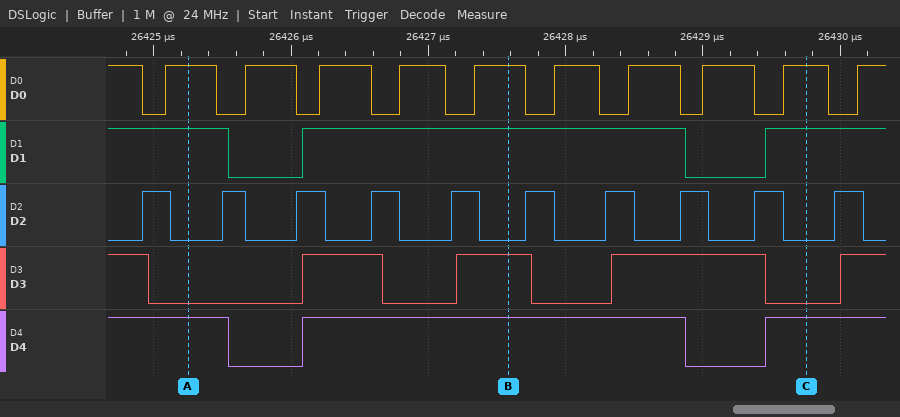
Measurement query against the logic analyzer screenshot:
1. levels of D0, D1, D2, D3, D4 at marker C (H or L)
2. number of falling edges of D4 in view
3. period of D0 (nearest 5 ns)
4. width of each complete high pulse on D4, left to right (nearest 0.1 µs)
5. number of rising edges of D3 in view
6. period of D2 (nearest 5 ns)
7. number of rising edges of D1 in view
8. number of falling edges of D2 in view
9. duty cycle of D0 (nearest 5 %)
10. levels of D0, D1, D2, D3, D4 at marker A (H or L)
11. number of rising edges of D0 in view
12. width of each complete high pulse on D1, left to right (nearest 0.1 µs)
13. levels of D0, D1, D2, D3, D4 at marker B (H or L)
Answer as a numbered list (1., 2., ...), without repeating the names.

1. D0=H, D1=H, D2=L, D3=L, D4=H
2. 2
3. 560 ns
4. 2.8 µs
5. 4
6. 560 ns
7. 2
8. 10
9. 65 %
10. D0=H, D1=H, D2=L, D3=L, D4=H
11. 10
12. 2.8 µs
13. D0=H, D1=H, D2=L, D3=H, D4=H
